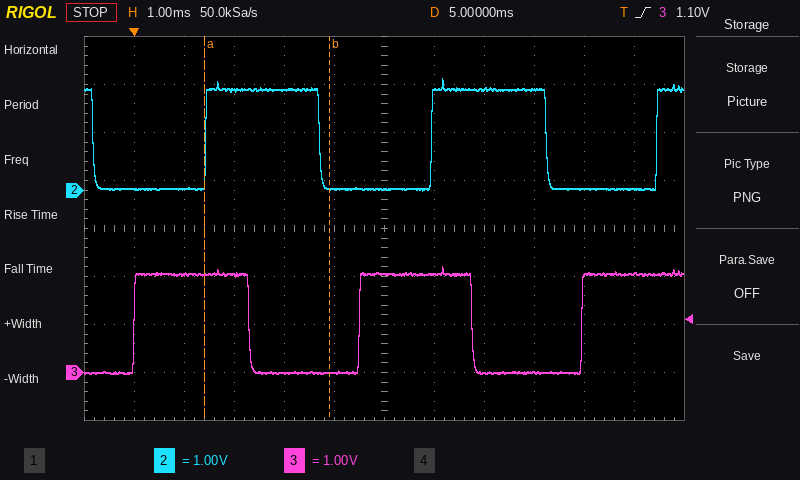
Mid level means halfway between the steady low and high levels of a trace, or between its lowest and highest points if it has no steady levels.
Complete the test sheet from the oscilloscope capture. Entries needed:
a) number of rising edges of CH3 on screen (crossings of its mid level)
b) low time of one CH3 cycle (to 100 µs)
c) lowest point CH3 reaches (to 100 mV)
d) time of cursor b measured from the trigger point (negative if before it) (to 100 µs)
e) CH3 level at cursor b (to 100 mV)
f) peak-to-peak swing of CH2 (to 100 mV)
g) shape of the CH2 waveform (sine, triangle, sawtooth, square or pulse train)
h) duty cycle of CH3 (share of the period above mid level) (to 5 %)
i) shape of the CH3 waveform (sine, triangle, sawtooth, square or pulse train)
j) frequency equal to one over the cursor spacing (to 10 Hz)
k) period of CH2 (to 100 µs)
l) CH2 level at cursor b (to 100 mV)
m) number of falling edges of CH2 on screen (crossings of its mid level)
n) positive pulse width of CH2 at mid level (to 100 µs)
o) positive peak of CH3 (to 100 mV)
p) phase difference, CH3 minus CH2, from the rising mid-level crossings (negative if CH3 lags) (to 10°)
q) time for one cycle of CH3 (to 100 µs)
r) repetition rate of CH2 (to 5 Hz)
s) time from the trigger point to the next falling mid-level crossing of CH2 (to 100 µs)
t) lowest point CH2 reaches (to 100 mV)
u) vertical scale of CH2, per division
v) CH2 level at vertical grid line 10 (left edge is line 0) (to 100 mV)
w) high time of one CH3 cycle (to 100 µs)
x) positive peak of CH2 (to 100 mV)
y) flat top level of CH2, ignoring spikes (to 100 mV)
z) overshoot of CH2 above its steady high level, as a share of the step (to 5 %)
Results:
3
2.2 ms
0.0 V
+3.9 ms
0.0 V
2.3 V
square
50 %
square
400 Hz
4.5 ms
0.0 V
3
2.3 ms
2.2 V
+120°
4.5 ms
220 Hz
3.7 ms
0.0 V
1 V
0.0 V
2.3 ms
2.3 V
2.1 V
10 %
